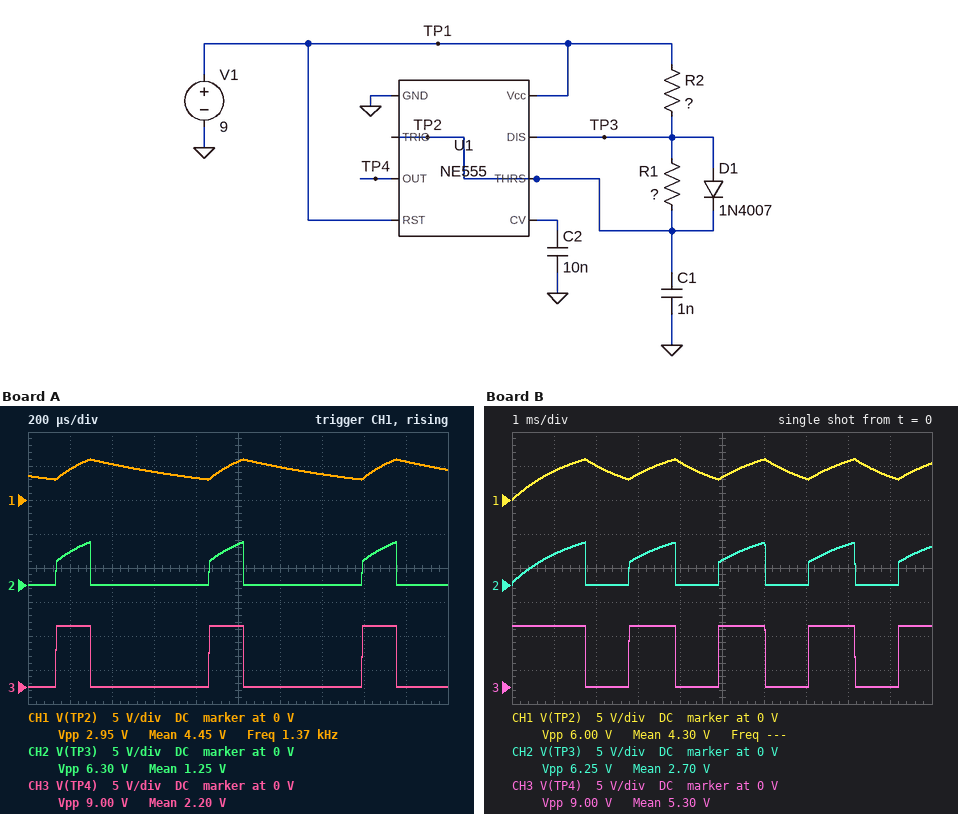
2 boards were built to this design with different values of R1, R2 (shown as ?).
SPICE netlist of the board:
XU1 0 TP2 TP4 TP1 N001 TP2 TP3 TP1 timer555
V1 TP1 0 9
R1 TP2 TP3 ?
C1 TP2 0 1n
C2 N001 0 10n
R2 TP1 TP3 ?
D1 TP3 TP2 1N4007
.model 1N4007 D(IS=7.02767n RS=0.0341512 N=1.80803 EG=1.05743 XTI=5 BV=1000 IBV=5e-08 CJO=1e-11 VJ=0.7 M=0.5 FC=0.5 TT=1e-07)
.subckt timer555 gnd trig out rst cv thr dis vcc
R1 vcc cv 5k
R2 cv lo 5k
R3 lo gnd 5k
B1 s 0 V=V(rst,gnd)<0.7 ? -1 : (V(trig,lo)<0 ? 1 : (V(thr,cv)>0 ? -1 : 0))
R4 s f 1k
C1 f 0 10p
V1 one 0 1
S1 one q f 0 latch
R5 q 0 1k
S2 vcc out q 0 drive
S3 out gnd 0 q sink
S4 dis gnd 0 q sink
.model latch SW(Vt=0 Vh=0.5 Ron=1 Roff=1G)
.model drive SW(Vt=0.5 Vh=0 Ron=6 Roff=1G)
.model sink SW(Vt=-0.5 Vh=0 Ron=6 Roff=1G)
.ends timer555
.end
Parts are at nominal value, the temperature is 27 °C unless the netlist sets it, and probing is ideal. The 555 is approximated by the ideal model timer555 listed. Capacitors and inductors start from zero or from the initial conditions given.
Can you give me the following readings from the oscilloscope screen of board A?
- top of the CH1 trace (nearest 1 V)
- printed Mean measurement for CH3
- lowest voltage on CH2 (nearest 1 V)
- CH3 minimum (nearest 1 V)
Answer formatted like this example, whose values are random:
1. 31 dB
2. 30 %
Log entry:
1. 6 V
2. 2.20 V
3. 0 V
4. 0 V
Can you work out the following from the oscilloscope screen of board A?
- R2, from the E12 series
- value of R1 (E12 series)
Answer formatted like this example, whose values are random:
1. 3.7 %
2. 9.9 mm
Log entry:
1. 220 kΩ
2. 820 kΩ
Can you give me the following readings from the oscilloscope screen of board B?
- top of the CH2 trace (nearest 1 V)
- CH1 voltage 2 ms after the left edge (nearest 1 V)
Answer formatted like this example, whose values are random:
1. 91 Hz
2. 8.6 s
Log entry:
1. 6 V
2. 5 V
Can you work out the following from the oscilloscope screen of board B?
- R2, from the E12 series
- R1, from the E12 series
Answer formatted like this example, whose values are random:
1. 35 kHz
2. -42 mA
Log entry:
1. 1.5 MΩ
2. 1.5 MΩ
